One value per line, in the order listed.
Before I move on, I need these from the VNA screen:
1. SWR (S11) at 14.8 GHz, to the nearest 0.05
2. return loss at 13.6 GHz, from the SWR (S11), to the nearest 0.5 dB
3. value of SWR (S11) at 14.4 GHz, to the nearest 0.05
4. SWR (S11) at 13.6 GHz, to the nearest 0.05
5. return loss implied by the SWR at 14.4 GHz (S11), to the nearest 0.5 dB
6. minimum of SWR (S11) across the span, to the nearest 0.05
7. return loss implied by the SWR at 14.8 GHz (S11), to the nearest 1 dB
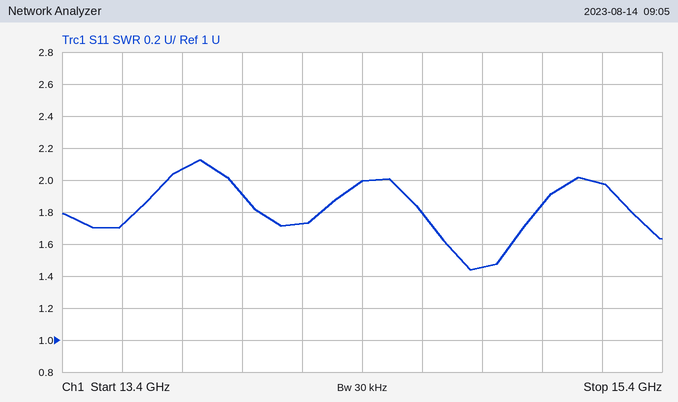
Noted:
1.45
11.5 dB
2.00
1.70
9.5 dB
1.45
15 dB
